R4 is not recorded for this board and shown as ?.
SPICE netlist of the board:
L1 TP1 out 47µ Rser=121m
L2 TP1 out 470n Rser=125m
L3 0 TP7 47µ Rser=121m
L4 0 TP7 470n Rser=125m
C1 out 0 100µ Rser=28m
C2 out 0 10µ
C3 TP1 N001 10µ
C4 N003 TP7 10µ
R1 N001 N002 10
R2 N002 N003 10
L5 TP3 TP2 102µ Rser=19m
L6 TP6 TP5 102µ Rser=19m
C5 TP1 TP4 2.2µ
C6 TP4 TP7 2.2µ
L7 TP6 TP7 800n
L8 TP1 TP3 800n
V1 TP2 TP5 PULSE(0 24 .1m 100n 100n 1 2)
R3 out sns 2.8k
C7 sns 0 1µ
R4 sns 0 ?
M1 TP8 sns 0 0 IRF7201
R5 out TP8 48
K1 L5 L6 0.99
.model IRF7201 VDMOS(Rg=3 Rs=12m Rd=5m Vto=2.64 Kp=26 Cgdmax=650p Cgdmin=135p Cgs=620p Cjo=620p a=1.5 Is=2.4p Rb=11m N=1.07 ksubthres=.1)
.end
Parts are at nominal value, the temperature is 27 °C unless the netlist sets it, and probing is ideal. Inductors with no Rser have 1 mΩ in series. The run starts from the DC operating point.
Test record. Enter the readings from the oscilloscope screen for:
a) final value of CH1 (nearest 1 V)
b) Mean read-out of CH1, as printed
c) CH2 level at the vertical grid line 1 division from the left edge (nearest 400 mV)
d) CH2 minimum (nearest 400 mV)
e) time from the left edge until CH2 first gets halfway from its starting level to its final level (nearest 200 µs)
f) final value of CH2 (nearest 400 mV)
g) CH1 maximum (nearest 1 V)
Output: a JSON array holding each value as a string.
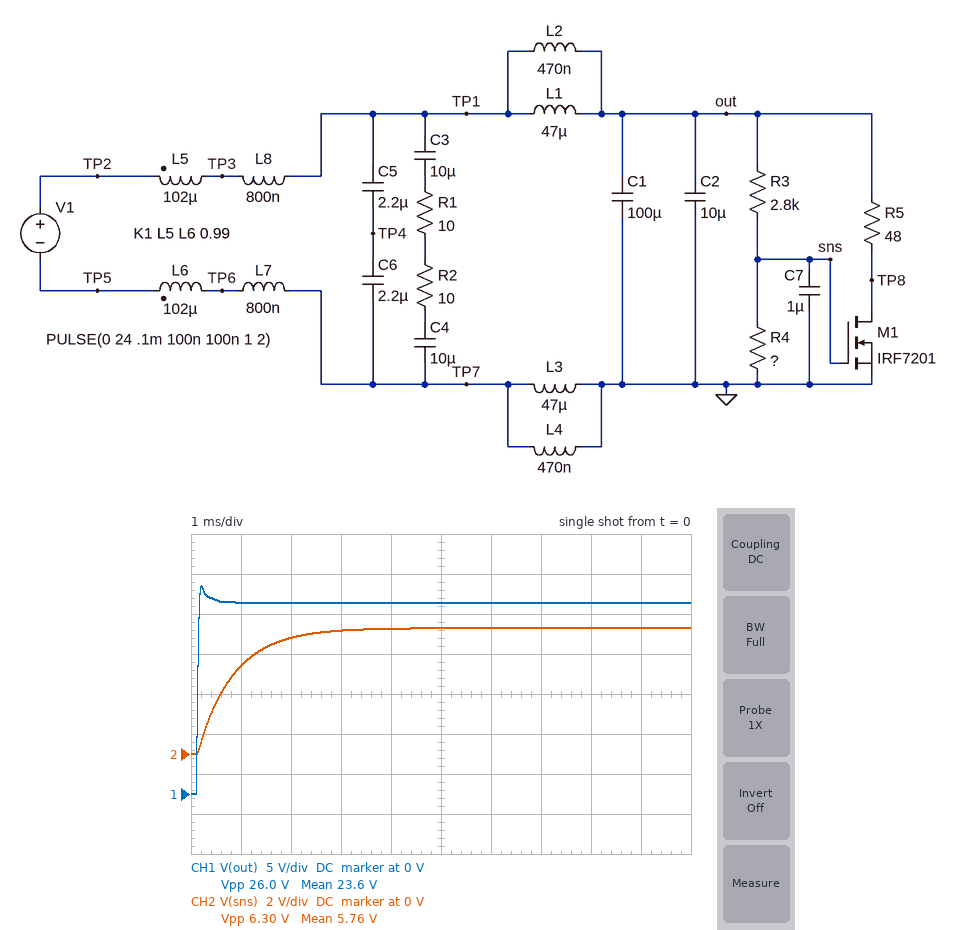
["24 V", "23.6 V", "4.4 V", "0 V", "600 µs", "6.4 V", "26 V"]
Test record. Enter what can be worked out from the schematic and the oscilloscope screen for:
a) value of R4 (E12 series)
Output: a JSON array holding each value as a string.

["1 kΩ"]
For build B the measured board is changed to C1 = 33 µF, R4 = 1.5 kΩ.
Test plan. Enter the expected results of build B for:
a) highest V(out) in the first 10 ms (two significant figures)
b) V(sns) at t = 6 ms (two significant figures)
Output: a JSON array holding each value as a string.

["29 V", "8.3 V"]
